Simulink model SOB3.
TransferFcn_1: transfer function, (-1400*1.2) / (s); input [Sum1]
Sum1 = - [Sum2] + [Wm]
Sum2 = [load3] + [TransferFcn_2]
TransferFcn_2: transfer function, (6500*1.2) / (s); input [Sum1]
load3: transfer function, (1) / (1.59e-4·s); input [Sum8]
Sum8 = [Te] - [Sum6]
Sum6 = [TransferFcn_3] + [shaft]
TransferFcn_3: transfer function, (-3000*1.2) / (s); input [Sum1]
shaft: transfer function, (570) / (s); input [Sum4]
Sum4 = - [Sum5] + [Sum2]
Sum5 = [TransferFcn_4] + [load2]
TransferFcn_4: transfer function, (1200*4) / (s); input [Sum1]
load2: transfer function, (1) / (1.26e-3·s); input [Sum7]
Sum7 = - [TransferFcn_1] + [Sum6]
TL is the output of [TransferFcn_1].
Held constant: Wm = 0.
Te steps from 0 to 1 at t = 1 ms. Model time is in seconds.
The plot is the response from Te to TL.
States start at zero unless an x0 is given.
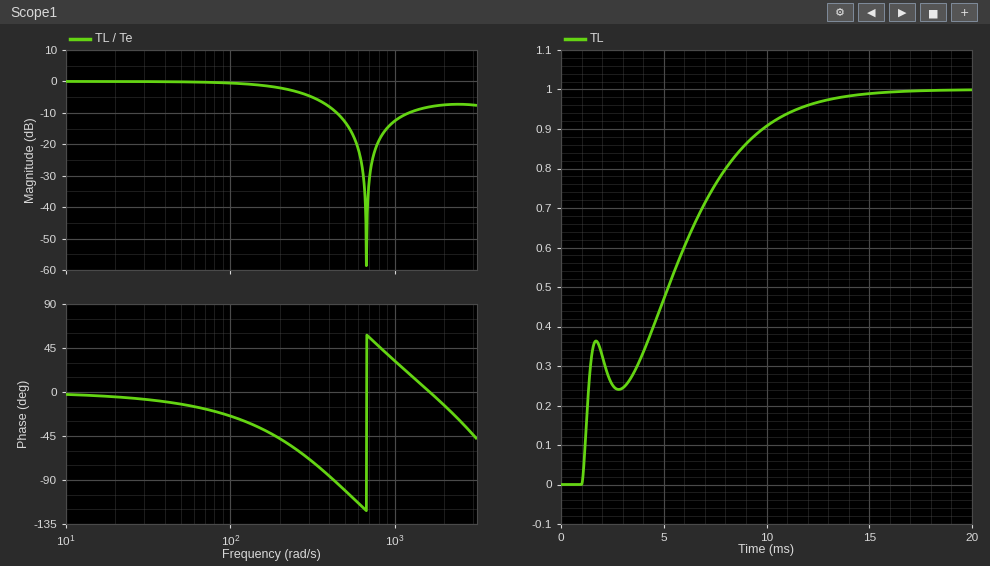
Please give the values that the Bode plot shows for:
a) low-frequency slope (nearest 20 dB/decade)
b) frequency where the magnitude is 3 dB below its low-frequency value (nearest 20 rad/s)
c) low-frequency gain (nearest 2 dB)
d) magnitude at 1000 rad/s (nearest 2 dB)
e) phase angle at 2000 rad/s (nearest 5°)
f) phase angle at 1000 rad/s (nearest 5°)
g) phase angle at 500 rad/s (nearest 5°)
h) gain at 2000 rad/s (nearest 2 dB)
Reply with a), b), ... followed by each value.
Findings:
a) 0 dB/decade
b) 240 rad/s
c) 0 dB
d) -12 dB
e) -15°
f) 30°
g) -100°
h) -8 dB
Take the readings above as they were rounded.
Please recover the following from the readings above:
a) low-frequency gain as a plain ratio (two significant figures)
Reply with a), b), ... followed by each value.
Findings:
a) 1.0
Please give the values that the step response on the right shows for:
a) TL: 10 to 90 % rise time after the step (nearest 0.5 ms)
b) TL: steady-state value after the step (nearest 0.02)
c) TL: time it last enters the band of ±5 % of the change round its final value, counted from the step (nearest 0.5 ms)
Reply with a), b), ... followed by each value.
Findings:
a) 8.5 ms
b) 1.00
c) 10.5 ms
